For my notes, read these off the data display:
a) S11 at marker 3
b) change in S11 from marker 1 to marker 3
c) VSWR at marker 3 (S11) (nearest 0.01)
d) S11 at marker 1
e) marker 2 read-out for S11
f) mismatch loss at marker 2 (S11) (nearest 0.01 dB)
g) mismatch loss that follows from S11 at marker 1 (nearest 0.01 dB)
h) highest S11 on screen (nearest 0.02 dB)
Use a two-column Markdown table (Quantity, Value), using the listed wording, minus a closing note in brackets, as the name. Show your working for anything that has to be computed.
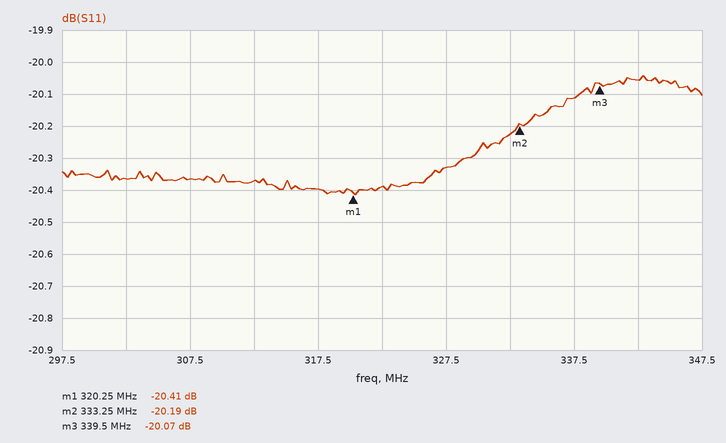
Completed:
| Quantity | Value |
|---|---|
| S11 at marker 3 | -20.07 dB |
| change in S11 from marker 1 to marker 3 | -20.07 − (-20.41) = 0.34 dB |
| VSWR at marker 3 (S11) | (1 + 0.0992)/(1 − 0.0992) ≈ 1.22 |
| S11 at marker 1 | -20.41 dB |
| marker 2 read-out for S11 | -20.19 dB |
| mismatch loss at marker 2 (S11) | −10 log10(1 − 10^(-20.19/10)) ≈ 0.04 dB |
| mismatch loss that follows from S11 at marker 1 | −10 log10(1 − 10^(-20.41/10)) ≈ 0.04 dB |
| highest S11 on screen | -20.04 dB |
